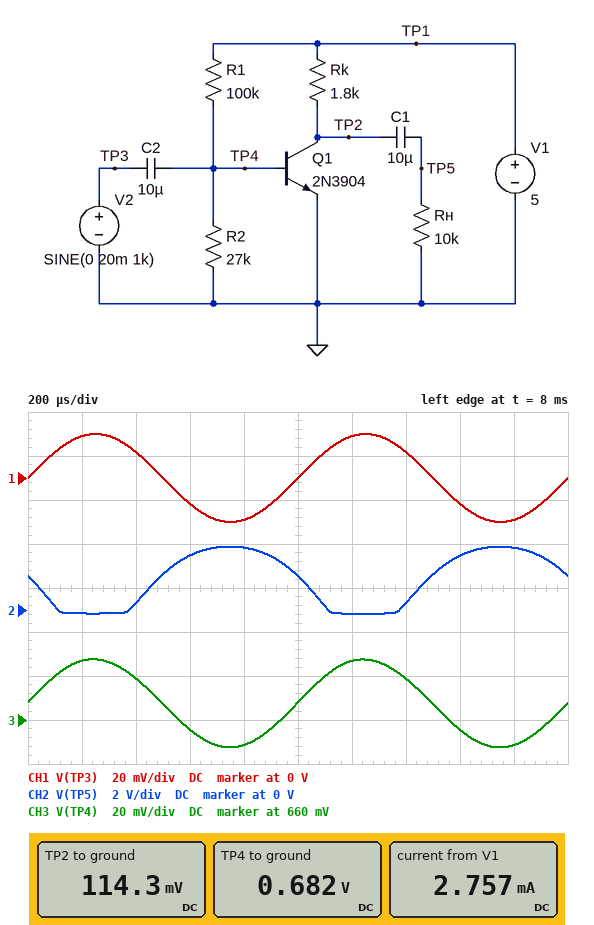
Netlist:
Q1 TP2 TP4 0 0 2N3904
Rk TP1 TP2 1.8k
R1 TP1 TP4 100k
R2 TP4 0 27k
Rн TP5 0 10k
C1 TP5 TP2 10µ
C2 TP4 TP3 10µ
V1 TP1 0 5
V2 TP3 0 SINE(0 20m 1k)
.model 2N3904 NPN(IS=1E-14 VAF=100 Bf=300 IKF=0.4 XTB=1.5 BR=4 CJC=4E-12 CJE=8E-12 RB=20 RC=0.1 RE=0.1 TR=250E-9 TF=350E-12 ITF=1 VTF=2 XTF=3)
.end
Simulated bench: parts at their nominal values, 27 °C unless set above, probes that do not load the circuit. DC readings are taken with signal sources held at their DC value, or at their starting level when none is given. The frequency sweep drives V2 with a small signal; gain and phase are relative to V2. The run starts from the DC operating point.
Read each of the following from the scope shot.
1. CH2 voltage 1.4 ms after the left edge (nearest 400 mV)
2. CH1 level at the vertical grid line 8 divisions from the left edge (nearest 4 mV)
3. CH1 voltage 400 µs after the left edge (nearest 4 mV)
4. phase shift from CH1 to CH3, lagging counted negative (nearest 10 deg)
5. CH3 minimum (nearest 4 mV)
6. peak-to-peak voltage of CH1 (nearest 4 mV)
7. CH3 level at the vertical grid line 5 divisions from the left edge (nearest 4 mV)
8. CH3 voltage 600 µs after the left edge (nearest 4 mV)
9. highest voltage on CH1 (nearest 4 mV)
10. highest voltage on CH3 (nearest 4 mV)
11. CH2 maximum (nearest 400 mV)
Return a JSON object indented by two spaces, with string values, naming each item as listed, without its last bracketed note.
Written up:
{
  "CH2 voltage 1.4 ms after the left edge": "400 mV",
  "CH1 level at the vertical grid line 8 divisions from the left edge": "-12 mV",
  "CH1 voltage 400 µs after the left edge": "12 mV",
  "phase shift from CH1 to CH3, lagging counted negative": "0 deg",
  "CH3 minimum": "648 mV",
  "peak-to-peak voltage of CH1": "40 mV",
  "CH3 level at the vertical grid line 5 divisions from the left edge": "668 mV",
  "CH3 voltage 600 µs after the left edge": "656 mV",
  "highest voltage on CH1": "20 mV",
  "highest voltage on CH3": "688 mV",
  "CH2 maximum": "2.8 V"
}
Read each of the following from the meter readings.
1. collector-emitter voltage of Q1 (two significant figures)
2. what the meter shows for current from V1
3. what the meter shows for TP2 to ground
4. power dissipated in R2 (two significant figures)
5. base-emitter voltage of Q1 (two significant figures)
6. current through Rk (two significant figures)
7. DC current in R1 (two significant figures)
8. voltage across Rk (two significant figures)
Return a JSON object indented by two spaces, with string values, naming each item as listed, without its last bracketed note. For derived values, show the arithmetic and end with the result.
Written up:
{
  "collector-emitter voltage of Q1": "114.3 mV = 110 mV",
  "what the meter shows for current from V1": "2.757 mA",
  "what the meter shows for TP2 to ground": "114.3 mV",
  "power dissipated in R2": "(682 mV)^2 / 27 kΩ = 17 µW",
  "base-emitter voltage of Q1": "682 mV = 680 mV",
  "current through Rk": "(5 V - 114.3 mV) / 1.8 kΩ = 2.7 mA",
  "DC current in R1": "(5 V - 682 mV) / 100 kΩ = 43 µA",
  "voltage across Rk": "5 V - 114.3 mV = 4.9 V"
}
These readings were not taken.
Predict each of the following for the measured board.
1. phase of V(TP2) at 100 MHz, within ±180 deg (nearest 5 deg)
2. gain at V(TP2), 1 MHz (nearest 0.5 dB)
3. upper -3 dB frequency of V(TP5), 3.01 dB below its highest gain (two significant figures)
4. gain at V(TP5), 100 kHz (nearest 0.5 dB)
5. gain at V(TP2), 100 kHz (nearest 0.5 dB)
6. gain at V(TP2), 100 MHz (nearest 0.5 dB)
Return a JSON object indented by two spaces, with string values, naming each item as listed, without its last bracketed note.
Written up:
{
  "phase of V(TP2) at 100 MHz, within ±180 deg": "15 deg",
  "gain at V(TP2), 1 MHz": "23.0 dB",
  "upper -3 dB frequency of V(TP5), 3.01 dB below its highest gain": "460 kHz",
  "gain at V(TP5), 100 kHz": "30.5 dB",
  "gain at V(TP2), 100 kHz": "30.5 dB",
  "gain at V(TP2), 100 MHz": "-9.0 dB"
}
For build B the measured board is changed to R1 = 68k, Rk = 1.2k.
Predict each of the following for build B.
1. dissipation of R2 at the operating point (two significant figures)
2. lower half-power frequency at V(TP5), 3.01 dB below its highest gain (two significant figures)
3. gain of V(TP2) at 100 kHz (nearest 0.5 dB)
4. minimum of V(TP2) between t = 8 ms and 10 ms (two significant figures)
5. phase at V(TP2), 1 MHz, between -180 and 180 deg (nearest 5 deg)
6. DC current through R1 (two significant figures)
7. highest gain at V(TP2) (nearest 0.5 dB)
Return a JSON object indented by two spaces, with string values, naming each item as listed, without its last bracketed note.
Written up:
{
  "dissipation of R2 at the operating point": "18 µW",
  "lower half-power frequency at V(TP5), 3.01 dB below its highest gain": "280 Hz",
  "gain of V(TP2) at 100 kHz": "25.0 dB",
  "minimum of V(TP2) between t = 8 ms and 10 ms": "55 mV",
  "phase at V(TP2), 1 MHz, between -180 and 180 deg": "105 deg",
  "DC current through R1": "63 µA",
  "highest gain at V(TP2)": "25.5 dB"
}
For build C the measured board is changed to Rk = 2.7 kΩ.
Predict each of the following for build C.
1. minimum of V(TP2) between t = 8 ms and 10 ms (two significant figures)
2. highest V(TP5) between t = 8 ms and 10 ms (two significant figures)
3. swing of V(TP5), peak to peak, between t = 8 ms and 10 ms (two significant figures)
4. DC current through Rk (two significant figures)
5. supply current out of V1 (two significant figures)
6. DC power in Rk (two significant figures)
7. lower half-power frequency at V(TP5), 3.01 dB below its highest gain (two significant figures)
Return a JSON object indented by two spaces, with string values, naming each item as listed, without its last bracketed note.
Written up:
{
  "minimum of V(TP2) between t = 8 ms and 10 ms": "49 mV",
  "highest V(TP5) between t = 8 ms and 10 ms": "2.6 V",
  "swing of V(TP5), peak to peak, between t = 8 ms and 10 ms": "2.8 V",
  "DC current through Rk": "1.8 mA",
  "supply current out of V1": "1.9 mA",
  "DC power in Rk": "8.9 mW",
  "lower half-power frequency at V(TP5), 3.01 dB below its highest gain": "160 Hz"
}
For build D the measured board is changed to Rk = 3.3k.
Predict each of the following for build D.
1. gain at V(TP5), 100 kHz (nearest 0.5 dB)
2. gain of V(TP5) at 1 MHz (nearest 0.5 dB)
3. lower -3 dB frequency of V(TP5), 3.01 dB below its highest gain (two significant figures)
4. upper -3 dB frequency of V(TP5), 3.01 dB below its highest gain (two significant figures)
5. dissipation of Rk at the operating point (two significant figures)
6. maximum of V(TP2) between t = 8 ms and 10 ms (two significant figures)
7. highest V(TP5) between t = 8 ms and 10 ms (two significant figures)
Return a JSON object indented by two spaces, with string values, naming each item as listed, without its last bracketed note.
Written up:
{
  "gain at V(TP5), 100 kHz": "24.0 dB",
  "gain of V(TP5) at 1 MHz": "17.0 dB",
  "lower -3 dB frequency of V(TP5), 3.01 dB below its highest gain": "140 Hz",
  "upper -3 dB frequency of V(TP5), 3.01 dB below its highest gain": "500 kHz",
  "dissipation of Rk at the operating point": "7.3 mW",
  "maximum of V(TP2) between t = 8 ms and 10 ms": "2.7 V",
  "highest V(TP5) between t = 8 ms and 10 ms": "2.5 V"
}
